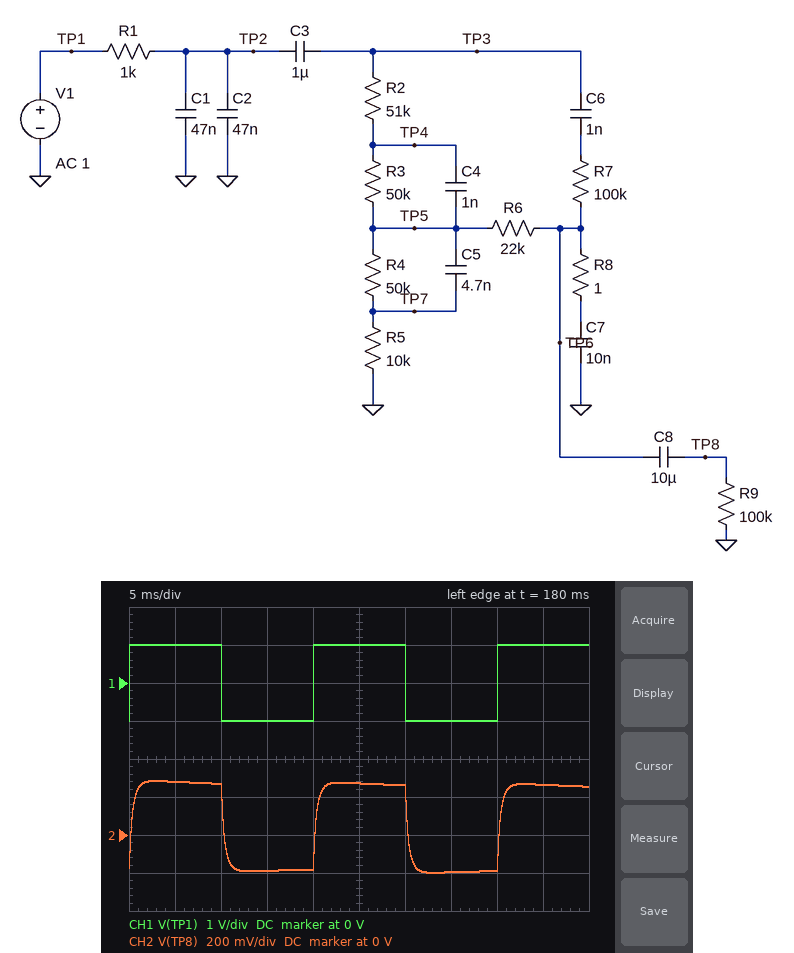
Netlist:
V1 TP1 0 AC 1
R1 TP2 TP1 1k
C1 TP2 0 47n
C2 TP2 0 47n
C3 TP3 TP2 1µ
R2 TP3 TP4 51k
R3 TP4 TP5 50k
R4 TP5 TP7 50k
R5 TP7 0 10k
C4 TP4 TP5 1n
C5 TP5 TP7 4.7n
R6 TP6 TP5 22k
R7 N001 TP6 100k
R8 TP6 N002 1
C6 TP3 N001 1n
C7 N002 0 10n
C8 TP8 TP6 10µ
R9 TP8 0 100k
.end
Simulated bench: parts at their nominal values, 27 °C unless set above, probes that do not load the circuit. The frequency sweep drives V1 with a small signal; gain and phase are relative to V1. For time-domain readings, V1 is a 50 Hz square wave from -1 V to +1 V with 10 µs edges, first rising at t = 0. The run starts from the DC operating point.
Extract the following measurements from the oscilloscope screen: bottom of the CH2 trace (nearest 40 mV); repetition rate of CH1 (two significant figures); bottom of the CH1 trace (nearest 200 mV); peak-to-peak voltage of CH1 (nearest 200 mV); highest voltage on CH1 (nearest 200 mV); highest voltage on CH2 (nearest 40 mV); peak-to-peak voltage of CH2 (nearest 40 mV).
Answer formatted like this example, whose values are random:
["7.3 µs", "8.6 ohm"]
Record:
["-200 mV", "50 Hz", "-1.0 V", "2.0 V", "1.0 V", "280 mV", "480 mV"]
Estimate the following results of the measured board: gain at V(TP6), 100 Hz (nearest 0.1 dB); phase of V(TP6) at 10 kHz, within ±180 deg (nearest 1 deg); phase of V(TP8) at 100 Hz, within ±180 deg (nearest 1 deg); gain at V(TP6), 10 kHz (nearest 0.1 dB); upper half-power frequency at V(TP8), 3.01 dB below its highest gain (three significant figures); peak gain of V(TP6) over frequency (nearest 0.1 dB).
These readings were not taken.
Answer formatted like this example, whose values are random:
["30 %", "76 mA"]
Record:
["-13.0 dB", "-159 deg", "-14 deg", "-48.1 dB", "398 Hz", "-12.7 dB"]
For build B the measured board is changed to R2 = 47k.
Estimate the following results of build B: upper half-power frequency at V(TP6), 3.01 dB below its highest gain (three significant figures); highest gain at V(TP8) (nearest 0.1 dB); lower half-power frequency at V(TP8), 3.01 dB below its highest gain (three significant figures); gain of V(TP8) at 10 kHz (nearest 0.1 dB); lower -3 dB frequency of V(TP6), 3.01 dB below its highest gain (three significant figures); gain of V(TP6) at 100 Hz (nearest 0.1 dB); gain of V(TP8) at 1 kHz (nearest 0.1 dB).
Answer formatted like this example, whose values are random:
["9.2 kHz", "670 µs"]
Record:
["397 Hz", "-12.5 dB", "1.16 Hz", "-47.9 dB", "1.14 Hz", "-12.8 dB", "-19.9 dB"]
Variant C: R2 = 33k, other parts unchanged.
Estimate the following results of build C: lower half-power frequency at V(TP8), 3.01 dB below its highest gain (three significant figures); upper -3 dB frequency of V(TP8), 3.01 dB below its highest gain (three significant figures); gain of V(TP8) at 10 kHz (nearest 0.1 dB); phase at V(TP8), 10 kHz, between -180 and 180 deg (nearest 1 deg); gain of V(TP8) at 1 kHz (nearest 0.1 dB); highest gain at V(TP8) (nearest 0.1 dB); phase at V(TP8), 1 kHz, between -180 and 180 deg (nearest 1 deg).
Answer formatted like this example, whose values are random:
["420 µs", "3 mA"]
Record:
["1.29 Hz", "395 Hz", "-47.1 dB", "-157 deg", "-19.2 dB", "-11.6 dB", "-74 deg"]
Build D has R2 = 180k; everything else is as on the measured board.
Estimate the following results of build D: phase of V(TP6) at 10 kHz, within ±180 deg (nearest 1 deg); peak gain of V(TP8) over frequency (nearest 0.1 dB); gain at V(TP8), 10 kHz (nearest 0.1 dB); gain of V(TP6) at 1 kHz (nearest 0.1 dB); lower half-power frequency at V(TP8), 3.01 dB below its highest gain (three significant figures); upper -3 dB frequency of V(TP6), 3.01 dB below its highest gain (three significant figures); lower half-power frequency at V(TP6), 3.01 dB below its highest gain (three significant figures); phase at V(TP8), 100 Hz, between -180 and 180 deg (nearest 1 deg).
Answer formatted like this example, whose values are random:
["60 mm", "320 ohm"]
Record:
["-159 deg", "-18.3 dB", "-50.4 dB", "-22.9 dB", "604 mHz", "638 Hz", "562 mHz", "-10 deg"]
